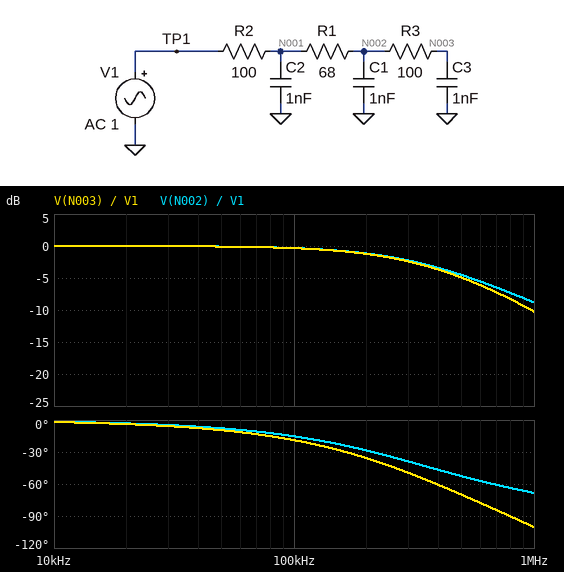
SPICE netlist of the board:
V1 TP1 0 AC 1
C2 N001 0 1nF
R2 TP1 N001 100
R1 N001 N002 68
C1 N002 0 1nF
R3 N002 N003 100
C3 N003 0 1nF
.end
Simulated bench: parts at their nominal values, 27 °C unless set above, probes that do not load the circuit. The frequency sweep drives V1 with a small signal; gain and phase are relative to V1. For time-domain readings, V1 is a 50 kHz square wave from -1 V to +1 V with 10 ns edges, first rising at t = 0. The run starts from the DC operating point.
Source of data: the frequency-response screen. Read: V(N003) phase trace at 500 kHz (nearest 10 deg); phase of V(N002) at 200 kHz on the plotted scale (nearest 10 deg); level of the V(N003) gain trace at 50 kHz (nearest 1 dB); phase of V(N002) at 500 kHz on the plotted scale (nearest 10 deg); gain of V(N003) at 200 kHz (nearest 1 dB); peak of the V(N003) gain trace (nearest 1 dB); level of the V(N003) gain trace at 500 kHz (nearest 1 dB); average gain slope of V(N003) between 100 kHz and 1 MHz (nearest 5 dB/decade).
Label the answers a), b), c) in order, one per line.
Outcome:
a) -70 deg
b) -30 deg
c) 0 dB
d) -50 deg
e) -1 dB
f) 0 dB
g) -5 dB
h) -10 dB/decade
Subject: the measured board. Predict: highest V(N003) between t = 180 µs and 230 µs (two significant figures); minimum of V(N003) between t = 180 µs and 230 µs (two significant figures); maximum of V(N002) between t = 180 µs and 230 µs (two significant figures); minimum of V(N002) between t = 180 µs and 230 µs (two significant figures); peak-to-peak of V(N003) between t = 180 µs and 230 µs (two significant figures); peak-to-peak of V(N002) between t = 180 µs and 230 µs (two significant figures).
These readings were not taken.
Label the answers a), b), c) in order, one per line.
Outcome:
a) 1.0 V
b) -1.0 V
c) 1.0 V
d) -1.0 V
e) 2.0 V
f) 2.0 V
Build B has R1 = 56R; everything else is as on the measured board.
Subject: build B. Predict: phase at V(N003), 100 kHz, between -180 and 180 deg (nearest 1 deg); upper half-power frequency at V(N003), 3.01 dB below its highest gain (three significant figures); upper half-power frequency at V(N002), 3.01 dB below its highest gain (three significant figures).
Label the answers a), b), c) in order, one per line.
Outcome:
a) -18 deg
b) 363 kHz
c) 383 kHz
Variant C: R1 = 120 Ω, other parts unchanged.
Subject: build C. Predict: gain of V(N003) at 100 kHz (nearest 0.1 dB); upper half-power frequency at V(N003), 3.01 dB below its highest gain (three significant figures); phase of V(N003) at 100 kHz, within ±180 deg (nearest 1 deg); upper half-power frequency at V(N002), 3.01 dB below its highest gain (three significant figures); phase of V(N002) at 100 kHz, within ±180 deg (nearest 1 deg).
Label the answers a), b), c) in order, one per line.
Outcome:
a) -0.5 dB
b) 289 kHz
c) -22 deg
d) 299 kHz
e) -19 deg
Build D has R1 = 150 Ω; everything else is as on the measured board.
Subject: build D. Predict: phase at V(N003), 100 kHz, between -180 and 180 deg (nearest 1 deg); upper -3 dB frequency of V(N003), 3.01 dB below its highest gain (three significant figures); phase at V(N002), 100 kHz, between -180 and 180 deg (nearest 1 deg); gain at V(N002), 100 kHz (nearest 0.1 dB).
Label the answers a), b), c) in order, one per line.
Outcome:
a) -24 deg
b) 263 kHz
c) -21 deg
d) -0.6 dB
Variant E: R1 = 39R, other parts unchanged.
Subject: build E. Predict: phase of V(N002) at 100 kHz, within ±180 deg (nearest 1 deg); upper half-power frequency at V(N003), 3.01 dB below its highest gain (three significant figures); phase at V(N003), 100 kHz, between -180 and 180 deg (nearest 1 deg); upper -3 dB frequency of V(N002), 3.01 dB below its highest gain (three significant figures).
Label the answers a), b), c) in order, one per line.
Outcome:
a) -13 deg
b) 387 kHz
c) -17 deg
d) 412 kHz
